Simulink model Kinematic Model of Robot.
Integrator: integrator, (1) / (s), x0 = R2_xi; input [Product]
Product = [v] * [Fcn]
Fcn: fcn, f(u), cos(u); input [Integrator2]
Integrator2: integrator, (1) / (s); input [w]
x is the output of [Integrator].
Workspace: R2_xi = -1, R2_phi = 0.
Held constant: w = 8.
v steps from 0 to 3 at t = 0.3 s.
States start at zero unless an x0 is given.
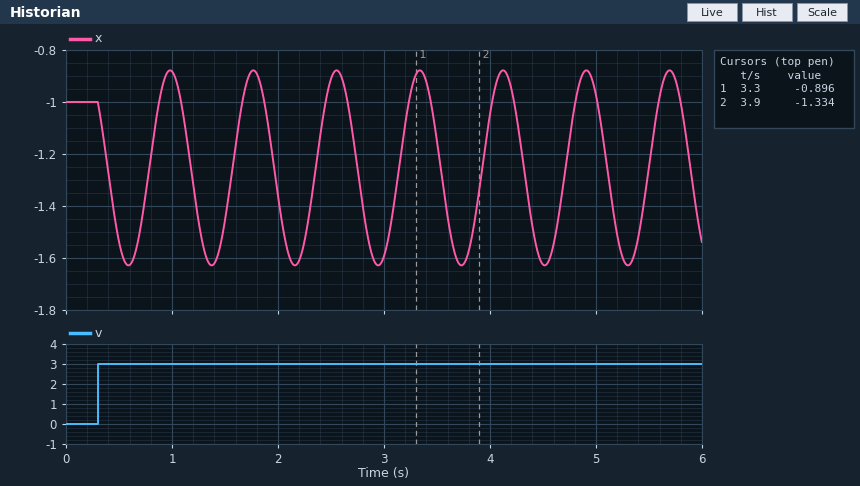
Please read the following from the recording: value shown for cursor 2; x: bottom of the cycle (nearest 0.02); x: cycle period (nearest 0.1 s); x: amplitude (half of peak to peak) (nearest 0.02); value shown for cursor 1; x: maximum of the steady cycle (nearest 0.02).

-1.334
-1.62
0.8 s
0.38
-0.896
-0.88
